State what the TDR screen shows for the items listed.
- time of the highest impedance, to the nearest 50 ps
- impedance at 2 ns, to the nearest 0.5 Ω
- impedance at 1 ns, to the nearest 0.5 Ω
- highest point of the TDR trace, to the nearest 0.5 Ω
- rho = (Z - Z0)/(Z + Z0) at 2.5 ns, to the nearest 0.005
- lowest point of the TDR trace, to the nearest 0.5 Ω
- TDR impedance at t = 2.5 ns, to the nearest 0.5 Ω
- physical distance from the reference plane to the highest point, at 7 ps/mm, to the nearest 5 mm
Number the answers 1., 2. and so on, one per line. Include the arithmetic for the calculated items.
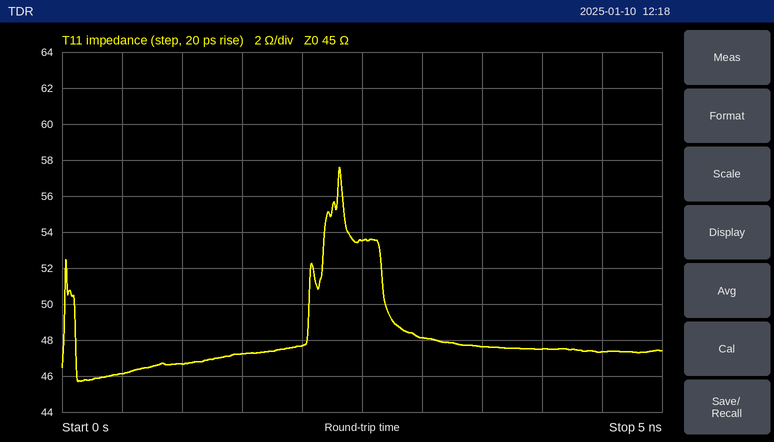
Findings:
1. 2.30 ns
2. 47.5 Ω
3. 46.5 Ω
4. 57.5 Ω
5. (53.5 − 45)/(53.5 + 45) ≈ +0.0863, so +0.085 to the nearest 0.005
6. 45.5 Ω
7. 53.5 Ω
8. 2.30 ns / 2 / 7 ps/mm ≈ 164 mm, so 165 mm to the nearest 5 mm
